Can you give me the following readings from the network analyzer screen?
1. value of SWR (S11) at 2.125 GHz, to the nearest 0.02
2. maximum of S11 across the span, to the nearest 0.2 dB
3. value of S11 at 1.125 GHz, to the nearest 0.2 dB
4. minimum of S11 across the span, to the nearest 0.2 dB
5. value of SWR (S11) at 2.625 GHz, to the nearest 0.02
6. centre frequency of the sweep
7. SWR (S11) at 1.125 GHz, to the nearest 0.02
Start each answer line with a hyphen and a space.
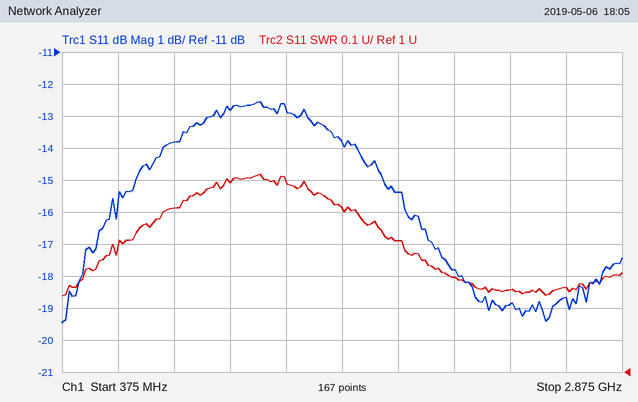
- 1.30
- -12.6 dB
- -12.8 dB
- -19.4 dB
- 1.26
- 1.625 GHz
- 1.60
